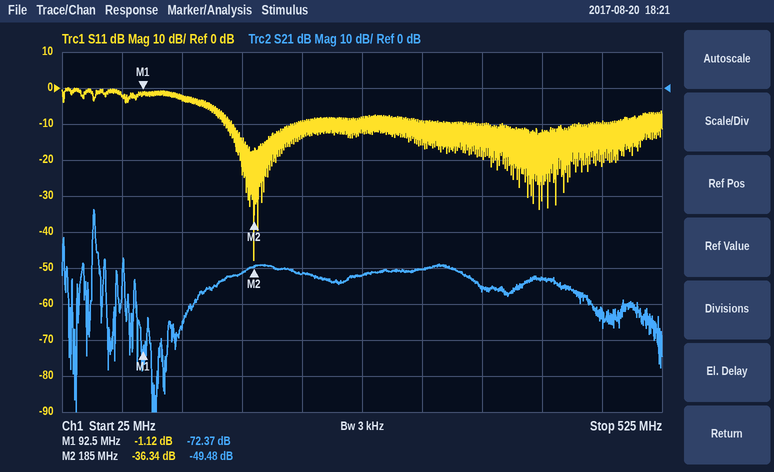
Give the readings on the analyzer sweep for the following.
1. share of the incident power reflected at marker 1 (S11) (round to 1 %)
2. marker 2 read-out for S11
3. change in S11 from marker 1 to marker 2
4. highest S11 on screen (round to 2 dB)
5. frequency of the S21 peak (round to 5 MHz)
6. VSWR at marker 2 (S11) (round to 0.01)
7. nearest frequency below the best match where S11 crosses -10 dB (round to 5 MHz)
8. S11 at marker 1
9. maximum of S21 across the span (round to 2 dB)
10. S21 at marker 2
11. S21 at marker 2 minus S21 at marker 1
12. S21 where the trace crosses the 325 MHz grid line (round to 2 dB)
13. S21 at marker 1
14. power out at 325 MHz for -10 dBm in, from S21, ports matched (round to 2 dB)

77 %
-36.34 dB
-35.22 dB
0 dB
50 MHz
1.03
165 MHz
-1.12 dB
-34 dB
-49.48 dB
22.89 dB
-50 dB
-72.37 dB
-60 dBm
